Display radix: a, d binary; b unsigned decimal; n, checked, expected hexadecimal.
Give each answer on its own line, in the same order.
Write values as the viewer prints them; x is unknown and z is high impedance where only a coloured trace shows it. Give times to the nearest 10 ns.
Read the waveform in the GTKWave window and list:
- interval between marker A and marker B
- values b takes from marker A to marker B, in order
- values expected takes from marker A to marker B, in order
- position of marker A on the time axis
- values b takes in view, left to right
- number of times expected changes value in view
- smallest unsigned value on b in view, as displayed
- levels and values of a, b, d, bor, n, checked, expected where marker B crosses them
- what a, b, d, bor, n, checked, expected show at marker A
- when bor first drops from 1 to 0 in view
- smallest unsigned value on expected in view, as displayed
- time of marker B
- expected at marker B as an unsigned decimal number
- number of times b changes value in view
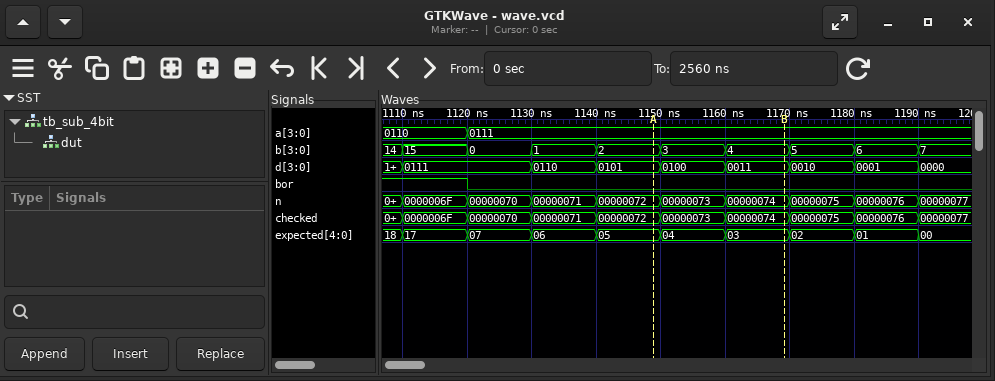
20 ns
2, 3, 4
05, 04, 03
1150 ns
14, 15, 0, 1, 2, 3, 4, 5, 6, 7
9
0
a=0111, b=4, d=0011, bor=0, n=00000074, checked=00000074, expected=03
a=0111, b=2, d=0101, bor=0, n=00000072, checked=00000072, expected=05
1120 ns
00
1170 ns
3
9
